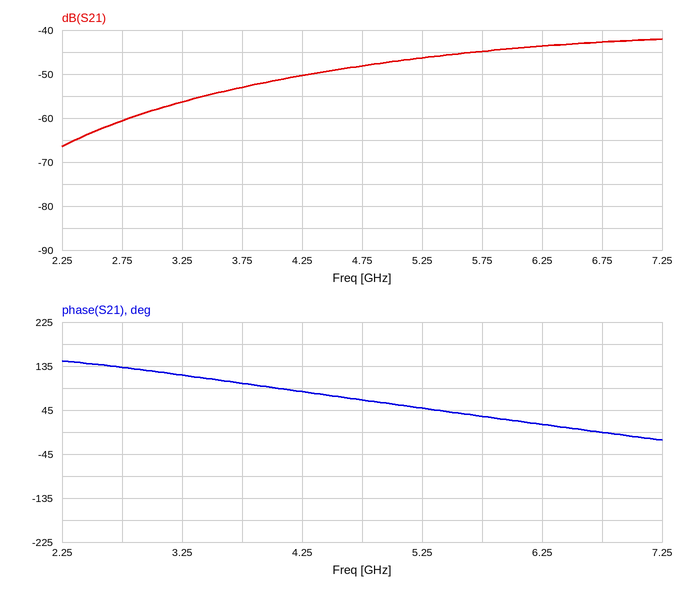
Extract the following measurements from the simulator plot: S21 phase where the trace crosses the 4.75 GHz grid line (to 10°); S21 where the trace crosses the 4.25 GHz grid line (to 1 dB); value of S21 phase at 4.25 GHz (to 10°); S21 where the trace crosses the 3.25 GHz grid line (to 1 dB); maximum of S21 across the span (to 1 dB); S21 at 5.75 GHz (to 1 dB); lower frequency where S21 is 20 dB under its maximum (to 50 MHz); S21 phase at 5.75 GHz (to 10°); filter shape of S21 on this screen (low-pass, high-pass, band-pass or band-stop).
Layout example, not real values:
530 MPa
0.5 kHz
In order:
70°
-50 dB
80°
-56 dB
-42 dB
-45 dB
2.60 GHz
30°
high-pass
